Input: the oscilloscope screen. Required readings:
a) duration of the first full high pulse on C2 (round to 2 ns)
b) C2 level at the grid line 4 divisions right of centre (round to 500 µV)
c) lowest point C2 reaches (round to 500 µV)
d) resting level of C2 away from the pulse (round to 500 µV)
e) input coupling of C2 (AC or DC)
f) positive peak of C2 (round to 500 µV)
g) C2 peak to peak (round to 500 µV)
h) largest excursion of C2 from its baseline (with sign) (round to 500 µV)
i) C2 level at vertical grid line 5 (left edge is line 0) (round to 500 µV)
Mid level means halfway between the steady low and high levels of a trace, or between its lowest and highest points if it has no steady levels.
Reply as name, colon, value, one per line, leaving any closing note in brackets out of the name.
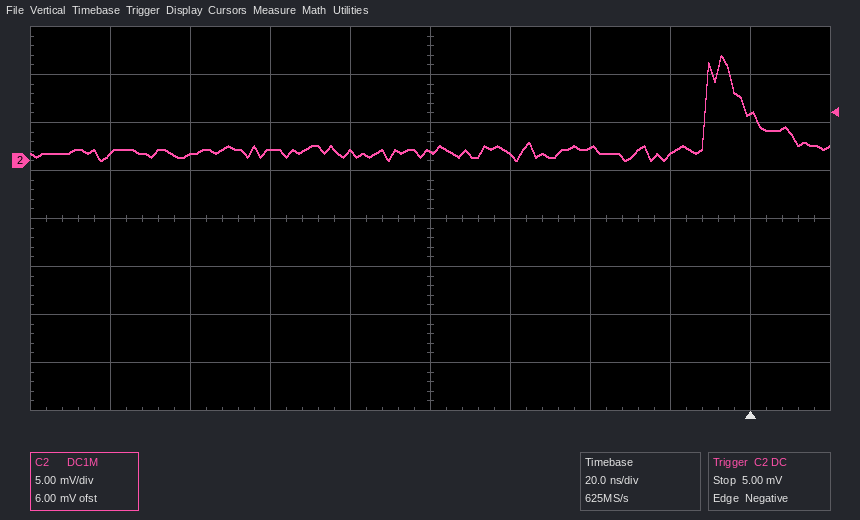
duration of the first full high pulse on C2: 10 ns
C2 level at the grid line 4 divisions right of centre: 5.0 mV
lowest point C2 reaches: 0.0 mV
resting level of C2 away from the pulse: 1.0 mV
input coupling of C2: DC
positive peak of C2: 11.0 mV
C2 peak to peak: 11.0 mV
largest excursion of C2 from its baseline (with sign): +10.0 mV
C2 level at vertical grid line 5 (left edge is line 0): 1.0 mV
